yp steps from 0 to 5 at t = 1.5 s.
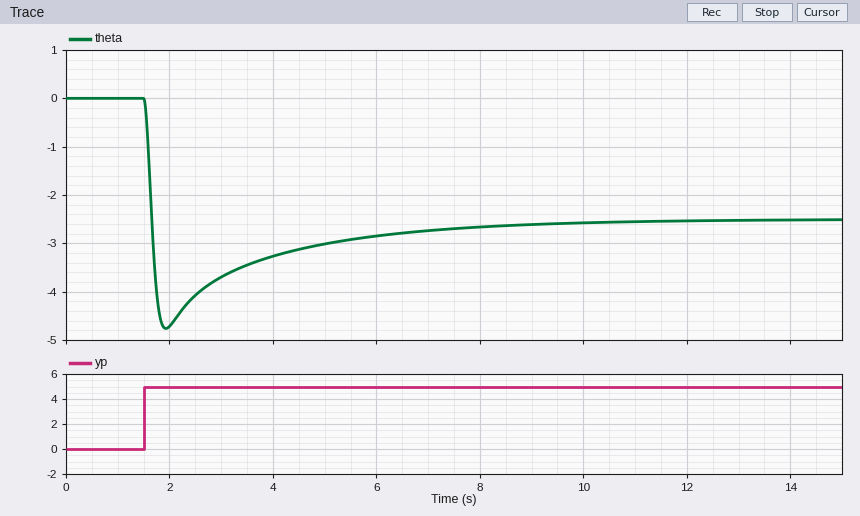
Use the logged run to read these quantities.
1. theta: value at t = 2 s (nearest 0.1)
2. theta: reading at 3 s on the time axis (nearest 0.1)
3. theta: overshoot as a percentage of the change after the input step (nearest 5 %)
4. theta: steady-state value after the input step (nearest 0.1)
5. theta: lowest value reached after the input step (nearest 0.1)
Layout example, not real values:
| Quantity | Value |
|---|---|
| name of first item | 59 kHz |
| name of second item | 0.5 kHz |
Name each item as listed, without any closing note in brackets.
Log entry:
| Quantity | Value |
|---|---|
| theta: value at t = 2 s | -4.7 |
| theta: reading at 3 s on the time axis | -3.7 |
| theta: overshoot as a percentage of the change after the input step | 90 % |
| theta: steady-state value after the input step | -2.5 |
| theta: lowest value reached after the input step | -4.8 |
